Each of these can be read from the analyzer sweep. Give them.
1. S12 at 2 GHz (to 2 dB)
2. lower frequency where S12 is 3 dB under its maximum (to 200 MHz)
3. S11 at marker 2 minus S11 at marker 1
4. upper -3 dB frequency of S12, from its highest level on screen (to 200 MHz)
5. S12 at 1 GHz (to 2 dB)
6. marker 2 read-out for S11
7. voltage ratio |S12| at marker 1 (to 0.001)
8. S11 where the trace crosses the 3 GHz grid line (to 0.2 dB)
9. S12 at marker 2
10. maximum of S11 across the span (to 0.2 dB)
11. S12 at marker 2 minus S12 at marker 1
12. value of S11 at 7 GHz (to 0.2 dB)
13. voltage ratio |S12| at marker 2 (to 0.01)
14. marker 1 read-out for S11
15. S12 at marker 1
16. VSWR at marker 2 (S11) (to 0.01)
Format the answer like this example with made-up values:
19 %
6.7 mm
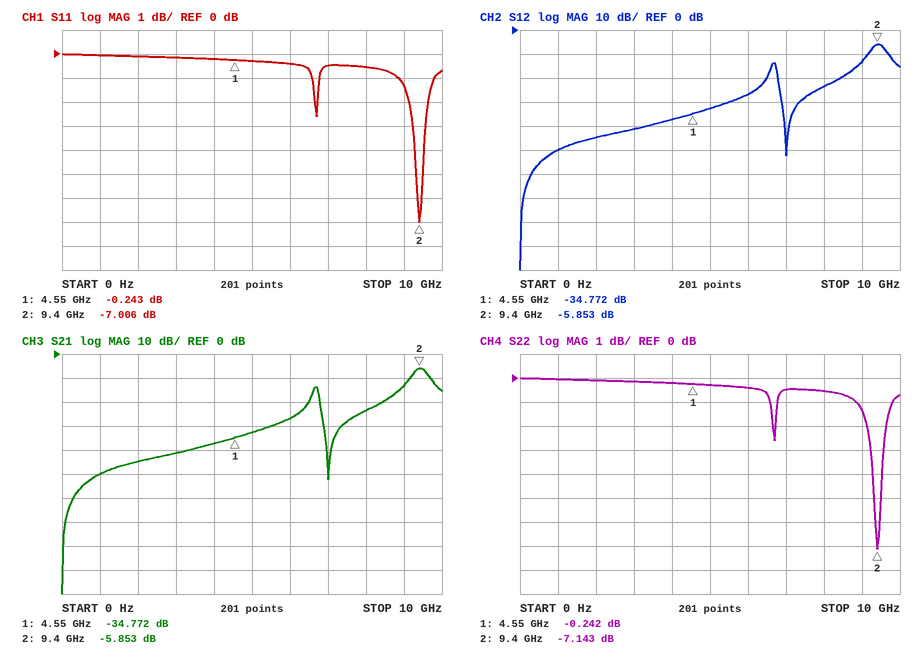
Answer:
-44 dB
9.2 GHz
-6.763 dB
9.6 GHz
-50 dB
-7.006 dB
0.018
-0.2 dB
-5.853 dB
0.0 dB
28.919 dB
-0.4 dB
0.51
-0.243 dB
-34.772 dB
2.61
